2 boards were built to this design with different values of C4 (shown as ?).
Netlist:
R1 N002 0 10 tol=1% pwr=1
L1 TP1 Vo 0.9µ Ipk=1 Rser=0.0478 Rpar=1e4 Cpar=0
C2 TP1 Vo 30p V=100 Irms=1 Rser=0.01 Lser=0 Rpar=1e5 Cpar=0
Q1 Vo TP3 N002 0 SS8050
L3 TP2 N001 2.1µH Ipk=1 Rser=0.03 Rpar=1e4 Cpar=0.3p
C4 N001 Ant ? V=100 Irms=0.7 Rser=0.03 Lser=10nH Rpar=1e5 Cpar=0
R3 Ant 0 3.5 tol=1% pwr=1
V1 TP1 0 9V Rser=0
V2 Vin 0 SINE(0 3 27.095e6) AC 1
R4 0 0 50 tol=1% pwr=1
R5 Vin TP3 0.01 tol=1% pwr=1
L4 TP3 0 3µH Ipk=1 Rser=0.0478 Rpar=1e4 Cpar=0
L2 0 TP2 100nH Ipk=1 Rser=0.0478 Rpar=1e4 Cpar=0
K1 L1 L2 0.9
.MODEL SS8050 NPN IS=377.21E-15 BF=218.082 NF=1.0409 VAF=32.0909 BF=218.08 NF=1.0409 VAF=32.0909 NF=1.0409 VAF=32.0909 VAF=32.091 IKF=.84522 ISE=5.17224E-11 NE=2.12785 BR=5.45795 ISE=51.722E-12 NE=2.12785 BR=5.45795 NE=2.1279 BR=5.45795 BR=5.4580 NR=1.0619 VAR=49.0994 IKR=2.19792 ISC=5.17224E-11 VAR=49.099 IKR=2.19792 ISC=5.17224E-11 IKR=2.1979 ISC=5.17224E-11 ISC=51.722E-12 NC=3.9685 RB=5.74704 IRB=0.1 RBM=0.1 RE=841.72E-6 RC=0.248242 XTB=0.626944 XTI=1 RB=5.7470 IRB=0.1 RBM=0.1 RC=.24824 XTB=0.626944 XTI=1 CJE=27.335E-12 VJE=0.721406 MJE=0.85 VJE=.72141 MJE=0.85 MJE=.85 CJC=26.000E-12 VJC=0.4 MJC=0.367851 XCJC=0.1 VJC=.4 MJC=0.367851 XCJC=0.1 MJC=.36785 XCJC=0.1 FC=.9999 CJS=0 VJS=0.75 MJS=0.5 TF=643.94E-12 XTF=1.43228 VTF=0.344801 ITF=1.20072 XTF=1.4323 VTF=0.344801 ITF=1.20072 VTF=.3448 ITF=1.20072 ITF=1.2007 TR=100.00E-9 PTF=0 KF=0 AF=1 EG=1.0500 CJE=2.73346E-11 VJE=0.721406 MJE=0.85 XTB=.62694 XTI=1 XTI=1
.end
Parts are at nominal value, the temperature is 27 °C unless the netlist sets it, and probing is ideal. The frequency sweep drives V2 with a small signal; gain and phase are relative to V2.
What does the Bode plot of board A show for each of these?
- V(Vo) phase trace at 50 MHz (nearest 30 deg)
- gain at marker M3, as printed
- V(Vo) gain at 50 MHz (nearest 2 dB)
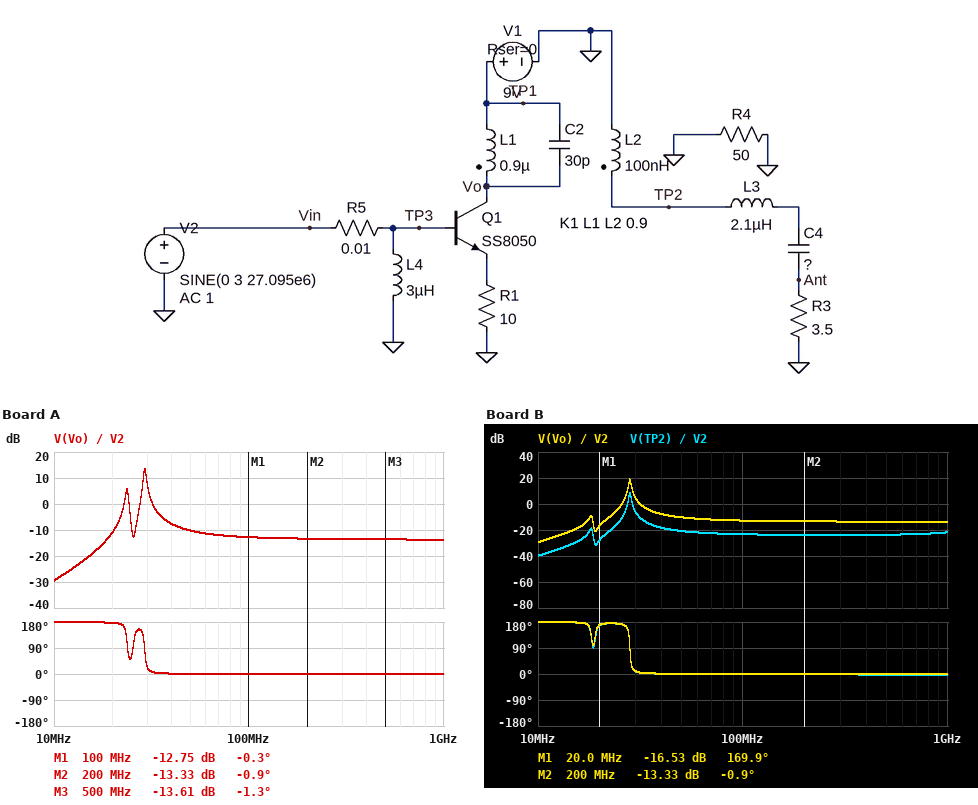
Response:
0 deg
-13.61 dB
-10 dB
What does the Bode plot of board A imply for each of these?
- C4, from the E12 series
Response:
18 pF
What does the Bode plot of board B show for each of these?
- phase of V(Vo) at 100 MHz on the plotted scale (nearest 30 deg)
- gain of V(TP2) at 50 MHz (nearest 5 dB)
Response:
0 deg
-20 dB
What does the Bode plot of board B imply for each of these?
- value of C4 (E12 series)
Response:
33 pF
